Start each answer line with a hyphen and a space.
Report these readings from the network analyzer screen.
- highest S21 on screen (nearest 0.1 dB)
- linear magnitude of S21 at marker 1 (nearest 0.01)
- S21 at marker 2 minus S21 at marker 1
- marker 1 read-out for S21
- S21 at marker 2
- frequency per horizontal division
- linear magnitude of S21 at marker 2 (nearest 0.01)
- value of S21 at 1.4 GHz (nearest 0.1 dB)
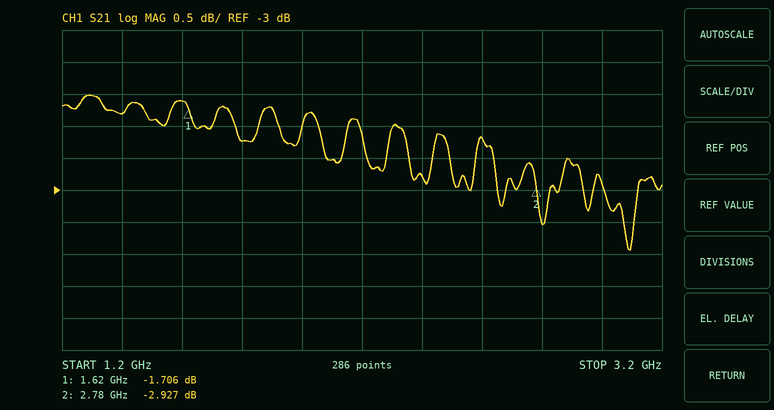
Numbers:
- -1.5 dB
- 0.82
- -1.221 dB
- -1.706 dB
- -2.927 dB
- 200 MHz
- 0.71
- -1.8 dB
